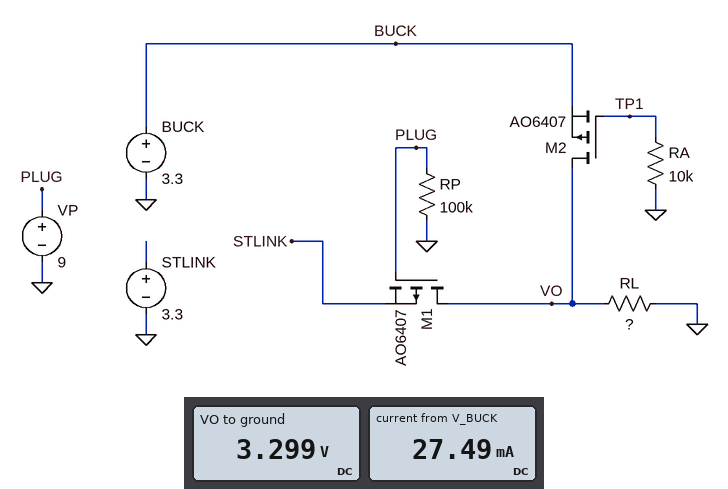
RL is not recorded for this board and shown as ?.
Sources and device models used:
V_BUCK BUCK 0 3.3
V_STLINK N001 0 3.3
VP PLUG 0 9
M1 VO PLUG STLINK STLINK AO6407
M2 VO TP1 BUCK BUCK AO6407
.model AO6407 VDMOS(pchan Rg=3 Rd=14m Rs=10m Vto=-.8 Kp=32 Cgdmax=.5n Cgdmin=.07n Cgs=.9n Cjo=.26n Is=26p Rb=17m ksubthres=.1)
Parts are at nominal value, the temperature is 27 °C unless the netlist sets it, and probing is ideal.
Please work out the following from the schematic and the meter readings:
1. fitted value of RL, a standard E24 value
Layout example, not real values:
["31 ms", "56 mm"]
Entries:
["120 Ω"]
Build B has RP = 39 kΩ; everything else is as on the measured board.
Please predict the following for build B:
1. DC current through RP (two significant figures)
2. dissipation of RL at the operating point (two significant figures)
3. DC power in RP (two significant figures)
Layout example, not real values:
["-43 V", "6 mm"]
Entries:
["230 µA", "91 mW", "2.1 mW"]
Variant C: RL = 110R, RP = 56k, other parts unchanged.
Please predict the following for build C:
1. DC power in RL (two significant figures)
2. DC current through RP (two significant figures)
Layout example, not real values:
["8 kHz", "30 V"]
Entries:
["99 mW", "160 µA"]
